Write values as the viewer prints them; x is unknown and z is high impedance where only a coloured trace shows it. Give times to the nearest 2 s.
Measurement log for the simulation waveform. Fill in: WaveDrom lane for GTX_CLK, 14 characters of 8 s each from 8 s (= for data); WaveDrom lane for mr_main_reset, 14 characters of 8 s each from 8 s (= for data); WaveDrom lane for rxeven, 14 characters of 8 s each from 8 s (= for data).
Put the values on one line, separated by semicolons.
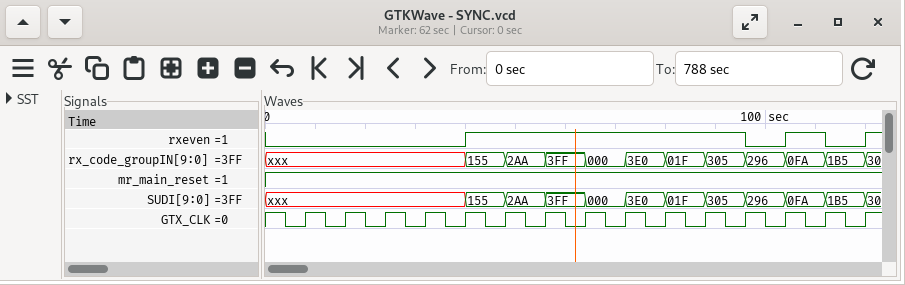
{name: 'GTX_CLK', wave: 'p.............'}; {name: 'mr_main_reset', wave: '1.............'}; {name: 'rxeven', wave: '0...1......010'}
